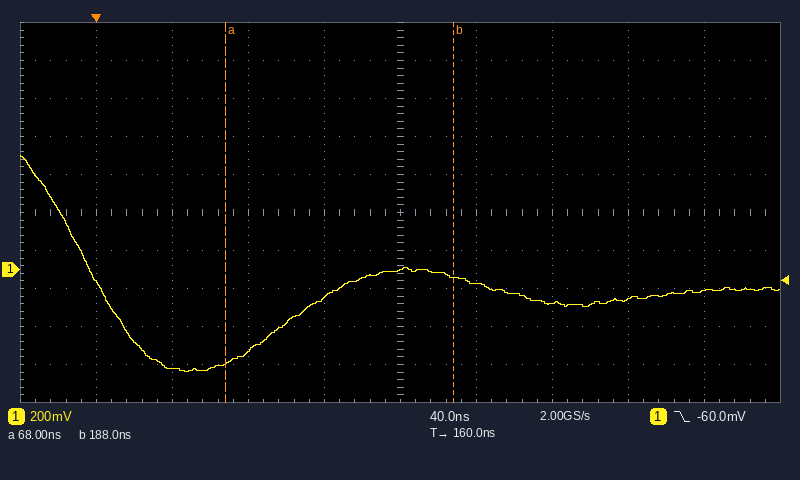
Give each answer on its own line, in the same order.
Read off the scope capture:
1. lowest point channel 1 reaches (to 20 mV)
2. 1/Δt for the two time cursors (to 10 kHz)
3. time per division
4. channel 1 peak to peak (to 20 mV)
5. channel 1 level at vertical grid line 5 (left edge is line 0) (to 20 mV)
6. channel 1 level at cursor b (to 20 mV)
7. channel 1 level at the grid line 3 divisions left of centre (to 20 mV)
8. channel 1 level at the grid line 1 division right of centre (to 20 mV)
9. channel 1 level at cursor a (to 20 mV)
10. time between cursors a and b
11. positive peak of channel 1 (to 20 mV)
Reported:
-540 mV
8.33 MHz
40 ns
1.14 V
0 mV
-40 mV
-520 mV
-80 mV
-500 mV
120 ns
600 mV
